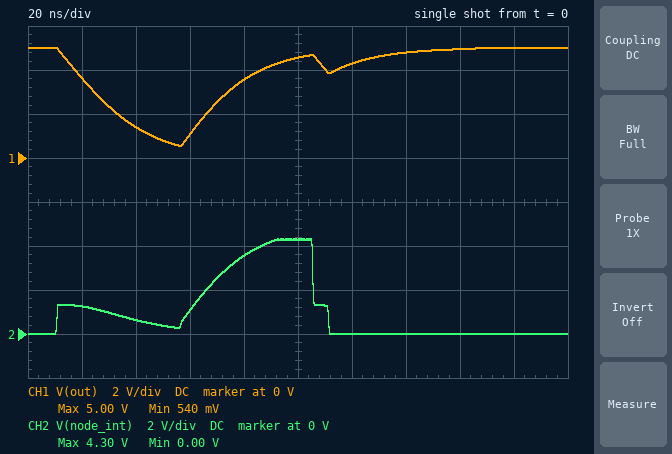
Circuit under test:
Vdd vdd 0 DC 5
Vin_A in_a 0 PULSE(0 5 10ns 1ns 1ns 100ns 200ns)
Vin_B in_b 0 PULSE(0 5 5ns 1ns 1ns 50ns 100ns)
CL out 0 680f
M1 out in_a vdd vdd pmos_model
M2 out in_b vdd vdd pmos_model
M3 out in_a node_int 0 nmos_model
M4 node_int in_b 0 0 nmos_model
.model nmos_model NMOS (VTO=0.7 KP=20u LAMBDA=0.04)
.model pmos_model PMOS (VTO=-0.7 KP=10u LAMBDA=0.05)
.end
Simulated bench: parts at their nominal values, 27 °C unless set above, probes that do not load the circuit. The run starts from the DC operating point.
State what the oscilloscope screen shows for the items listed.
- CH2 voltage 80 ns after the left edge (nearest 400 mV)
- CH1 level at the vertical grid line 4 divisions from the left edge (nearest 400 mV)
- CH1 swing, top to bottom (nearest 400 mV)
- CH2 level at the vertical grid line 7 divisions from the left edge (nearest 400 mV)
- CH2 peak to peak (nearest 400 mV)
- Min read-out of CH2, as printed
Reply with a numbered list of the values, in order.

1. 3.6 V
2. 3.6 V
3. 4.4 V
4. 0 V
5. 4.4 V
6. 0.00 V
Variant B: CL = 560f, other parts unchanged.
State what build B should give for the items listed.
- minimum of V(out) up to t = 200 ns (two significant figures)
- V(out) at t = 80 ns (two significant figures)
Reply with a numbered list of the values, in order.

1. 300 mV
2. 3.8 V
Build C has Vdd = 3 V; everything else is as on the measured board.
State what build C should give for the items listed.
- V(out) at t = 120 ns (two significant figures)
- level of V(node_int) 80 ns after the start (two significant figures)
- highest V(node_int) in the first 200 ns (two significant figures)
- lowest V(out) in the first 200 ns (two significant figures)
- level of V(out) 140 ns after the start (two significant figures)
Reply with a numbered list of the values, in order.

1. 1.8 V
2. 1.2 V
3. 2.1 V
4. 230 mV
5. 2.3 V
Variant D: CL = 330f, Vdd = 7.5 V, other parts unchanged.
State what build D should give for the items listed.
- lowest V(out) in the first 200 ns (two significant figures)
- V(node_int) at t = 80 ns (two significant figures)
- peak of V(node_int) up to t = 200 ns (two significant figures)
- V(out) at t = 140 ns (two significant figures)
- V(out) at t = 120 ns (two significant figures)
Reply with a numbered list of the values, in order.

1. 1.3 V
2. 4.3 V
3. 4.3 V
4. 7.5 V
5. 7.3 V
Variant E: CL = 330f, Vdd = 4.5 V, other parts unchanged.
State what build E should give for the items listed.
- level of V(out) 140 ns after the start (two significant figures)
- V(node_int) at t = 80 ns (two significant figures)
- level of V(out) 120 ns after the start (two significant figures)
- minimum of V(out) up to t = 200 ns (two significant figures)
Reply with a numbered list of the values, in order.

1. 4.4 V
2. 4.0 V
3. 3.8 V
4. 22 mV
